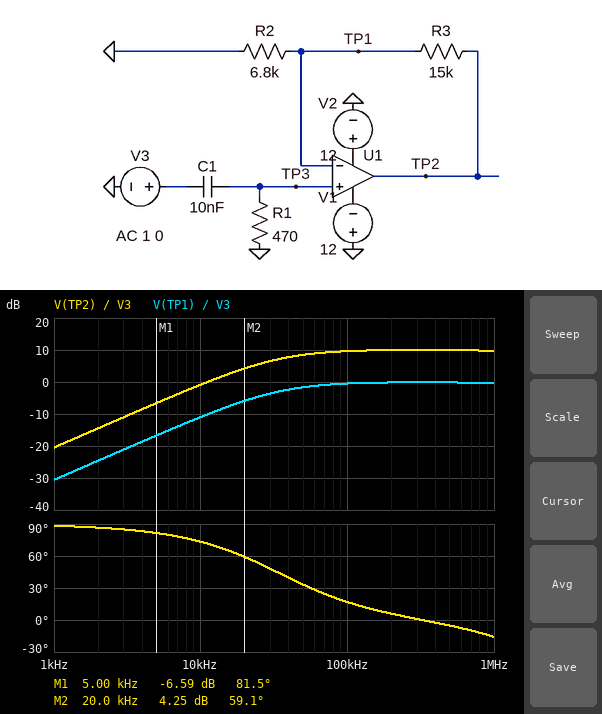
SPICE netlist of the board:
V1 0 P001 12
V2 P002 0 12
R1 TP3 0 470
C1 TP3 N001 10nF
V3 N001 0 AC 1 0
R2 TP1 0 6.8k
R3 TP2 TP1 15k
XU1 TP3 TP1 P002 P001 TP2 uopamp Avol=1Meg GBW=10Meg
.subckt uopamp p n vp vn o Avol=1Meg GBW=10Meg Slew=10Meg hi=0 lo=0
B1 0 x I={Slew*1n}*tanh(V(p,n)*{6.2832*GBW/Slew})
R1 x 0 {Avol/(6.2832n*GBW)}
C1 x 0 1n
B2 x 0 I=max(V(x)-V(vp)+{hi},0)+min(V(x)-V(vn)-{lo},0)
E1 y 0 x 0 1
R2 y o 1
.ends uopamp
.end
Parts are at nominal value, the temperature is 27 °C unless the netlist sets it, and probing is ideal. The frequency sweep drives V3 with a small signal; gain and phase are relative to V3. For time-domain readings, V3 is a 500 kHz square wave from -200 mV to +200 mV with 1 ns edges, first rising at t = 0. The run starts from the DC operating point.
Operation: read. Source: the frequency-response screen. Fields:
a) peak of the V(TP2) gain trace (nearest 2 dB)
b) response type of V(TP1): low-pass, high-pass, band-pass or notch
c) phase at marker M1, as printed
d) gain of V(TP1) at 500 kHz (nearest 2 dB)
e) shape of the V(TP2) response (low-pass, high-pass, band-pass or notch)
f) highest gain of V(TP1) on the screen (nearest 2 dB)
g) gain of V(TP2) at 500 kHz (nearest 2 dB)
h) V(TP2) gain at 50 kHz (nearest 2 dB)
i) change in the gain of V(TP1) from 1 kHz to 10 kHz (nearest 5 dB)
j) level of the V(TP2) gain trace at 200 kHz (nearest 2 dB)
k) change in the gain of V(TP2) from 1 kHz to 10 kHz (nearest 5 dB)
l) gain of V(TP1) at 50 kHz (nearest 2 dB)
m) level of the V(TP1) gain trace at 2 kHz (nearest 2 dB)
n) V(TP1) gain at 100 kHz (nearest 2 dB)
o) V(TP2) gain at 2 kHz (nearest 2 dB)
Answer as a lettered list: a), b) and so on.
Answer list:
a) 10 dB
b) high-pass
c) 81.5 deg
d) 0 dB
e) high-pass
f) 0 dB
g) 10 dB
h) 8 dB
i) 20 dB
j) 10 dB
k) 20 dB
l) -2 dB
m) -24 dB
n) 0 dB
o) -14 dB
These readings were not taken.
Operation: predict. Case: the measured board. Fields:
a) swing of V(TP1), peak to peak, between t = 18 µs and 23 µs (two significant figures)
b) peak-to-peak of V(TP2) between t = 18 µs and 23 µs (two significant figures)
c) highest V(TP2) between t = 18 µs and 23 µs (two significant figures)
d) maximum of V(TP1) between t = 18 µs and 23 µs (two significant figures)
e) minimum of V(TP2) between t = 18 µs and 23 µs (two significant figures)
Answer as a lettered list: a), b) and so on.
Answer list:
a) 420 mV
b) 1.3 V
c) 680 mV
d) 210 mV
e) -660 mV
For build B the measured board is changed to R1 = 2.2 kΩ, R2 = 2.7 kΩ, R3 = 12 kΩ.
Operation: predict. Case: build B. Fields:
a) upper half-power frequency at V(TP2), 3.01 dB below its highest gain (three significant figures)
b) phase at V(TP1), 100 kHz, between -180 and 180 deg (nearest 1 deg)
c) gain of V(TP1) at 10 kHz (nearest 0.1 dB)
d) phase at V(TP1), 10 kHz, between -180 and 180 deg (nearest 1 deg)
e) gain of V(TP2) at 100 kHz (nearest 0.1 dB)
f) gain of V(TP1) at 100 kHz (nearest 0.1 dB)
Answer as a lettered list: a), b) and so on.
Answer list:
a) 1.85 MHz
b) 1 deg
c) -1.8 dB
d) 36 deg
e) 14.7 dB
f) 0 dB
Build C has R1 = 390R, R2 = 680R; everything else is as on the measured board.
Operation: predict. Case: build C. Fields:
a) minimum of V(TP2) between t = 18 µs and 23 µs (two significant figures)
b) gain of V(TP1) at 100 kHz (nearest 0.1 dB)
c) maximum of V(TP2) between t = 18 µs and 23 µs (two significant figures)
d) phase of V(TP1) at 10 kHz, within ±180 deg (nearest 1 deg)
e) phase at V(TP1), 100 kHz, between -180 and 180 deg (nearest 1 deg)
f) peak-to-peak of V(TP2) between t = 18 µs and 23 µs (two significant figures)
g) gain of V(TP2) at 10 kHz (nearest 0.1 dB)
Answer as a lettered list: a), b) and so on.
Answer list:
a) -3.3 V
b) -0.9 dB
c) 3.4 V
d) 75 deg
e) 9 deg
f) 6.7 V
g) 14.8 dB
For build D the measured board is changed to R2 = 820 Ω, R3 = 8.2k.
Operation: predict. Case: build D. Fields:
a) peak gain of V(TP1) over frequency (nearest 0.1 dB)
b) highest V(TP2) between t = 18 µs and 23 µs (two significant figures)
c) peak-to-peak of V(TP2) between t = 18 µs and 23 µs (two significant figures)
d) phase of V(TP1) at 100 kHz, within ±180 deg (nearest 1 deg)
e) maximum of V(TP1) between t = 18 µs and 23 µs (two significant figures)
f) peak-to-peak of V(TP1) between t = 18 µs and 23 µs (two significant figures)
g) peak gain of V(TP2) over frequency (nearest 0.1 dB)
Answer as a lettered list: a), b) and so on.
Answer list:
a) -0.3 dB
b) 2.1 V
c) 4.1 V
d) 12 deg
e) 190 mV
f) 370 mV
g) 20.5 dB
